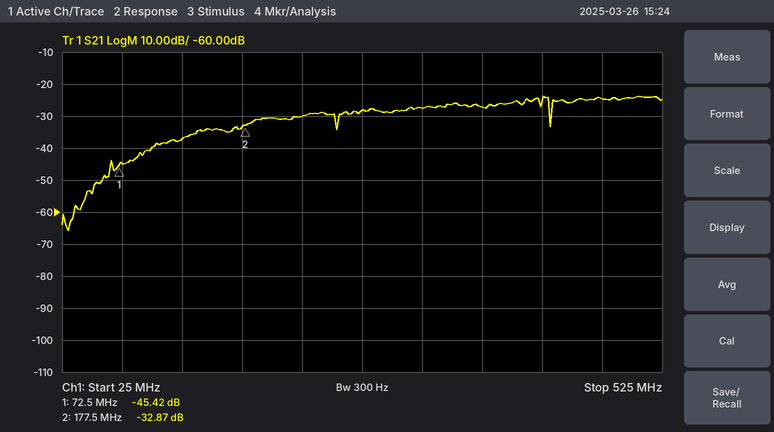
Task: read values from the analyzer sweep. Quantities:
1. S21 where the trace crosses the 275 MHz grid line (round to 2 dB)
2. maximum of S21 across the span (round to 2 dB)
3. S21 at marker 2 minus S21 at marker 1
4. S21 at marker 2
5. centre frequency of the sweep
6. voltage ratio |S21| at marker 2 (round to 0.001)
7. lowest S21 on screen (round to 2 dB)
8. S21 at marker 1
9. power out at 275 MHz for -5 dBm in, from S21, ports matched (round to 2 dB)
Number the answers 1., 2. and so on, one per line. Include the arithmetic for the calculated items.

1. -28 dB
2. -24 dB
3. -32.87 − (-45.42) = 12.55 dB
4. -32.87 dB
5. 275 MHz
6. 10^(-32.87/20) ≈ 0.023
7. -66 dB
8. -45.42 dB
9. -5 dBm + (-28 dB) = -34 dBm
